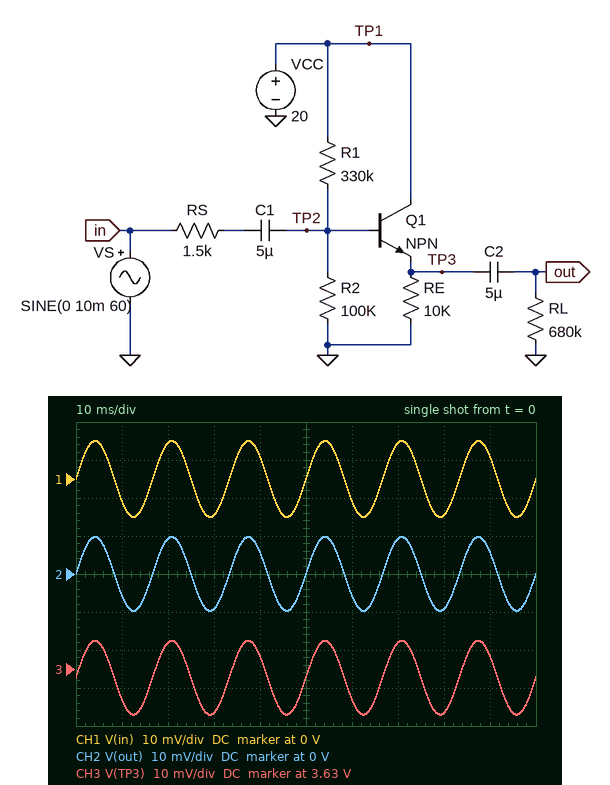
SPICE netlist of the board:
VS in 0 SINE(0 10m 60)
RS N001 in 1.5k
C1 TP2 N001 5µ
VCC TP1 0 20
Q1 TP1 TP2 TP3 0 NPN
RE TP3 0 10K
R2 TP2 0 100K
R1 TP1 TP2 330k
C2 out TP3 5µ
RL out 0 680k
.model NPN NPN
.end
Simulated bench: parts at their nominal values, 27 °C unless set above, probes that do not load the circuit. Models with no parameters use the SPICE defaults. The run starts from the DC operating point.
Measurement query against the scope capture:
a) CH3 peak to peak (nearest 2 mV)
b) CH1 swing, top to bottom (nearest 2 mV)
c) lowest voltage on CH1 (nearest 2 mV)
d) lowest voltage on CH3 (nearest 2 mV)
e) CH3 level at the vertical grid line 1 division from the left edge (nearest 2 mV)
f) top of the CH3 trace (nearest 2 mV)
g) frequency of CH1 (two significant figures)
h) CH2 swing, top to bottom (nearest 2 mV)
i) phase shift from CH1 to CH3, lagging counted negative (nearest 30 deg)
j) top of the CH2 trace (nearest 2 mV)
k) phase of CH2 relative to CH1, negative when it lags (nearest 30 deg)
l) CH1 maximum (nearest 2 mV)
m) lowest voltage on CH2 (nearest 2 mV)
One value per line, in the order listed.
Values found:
20 mV
20 mV
-10 mV
3.618 V
3.622 V
3.638 V
60 Hz
20 mV
0 deg
10 mV
0 deg
10 mV
-10 mV
